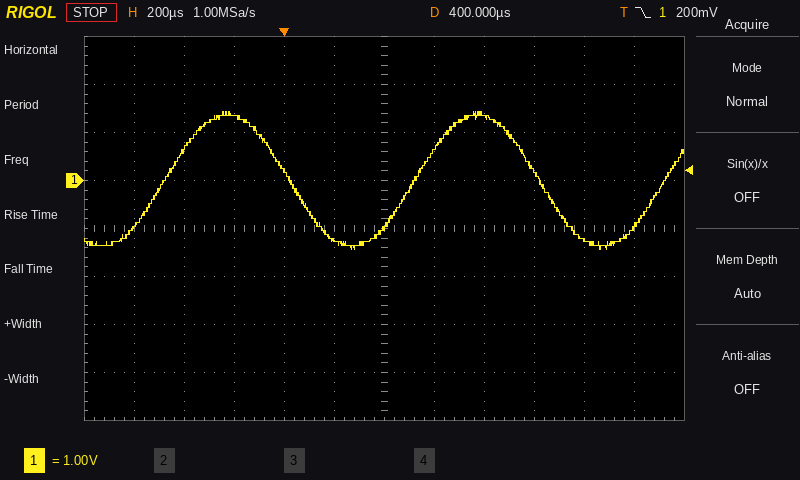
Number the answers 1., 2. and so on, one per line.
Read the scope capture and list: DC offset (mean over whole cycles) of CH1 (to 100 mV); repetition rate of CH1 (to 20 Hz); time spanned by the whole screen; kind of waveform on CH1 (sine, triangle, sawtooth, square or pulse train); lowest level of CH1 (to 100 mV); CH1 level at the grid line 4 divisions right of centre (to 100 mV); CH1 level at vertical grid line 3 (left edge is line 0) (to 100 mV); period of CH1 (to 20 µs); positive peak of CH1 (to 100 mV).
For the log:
1. 0.0 V
2. 1.00 kHz
3. 2.4 ms
4. sine
5. -1.4 V
6. -1.2 V
7. 1.4 V
8. 1.00 ms
9. 1.4 V
